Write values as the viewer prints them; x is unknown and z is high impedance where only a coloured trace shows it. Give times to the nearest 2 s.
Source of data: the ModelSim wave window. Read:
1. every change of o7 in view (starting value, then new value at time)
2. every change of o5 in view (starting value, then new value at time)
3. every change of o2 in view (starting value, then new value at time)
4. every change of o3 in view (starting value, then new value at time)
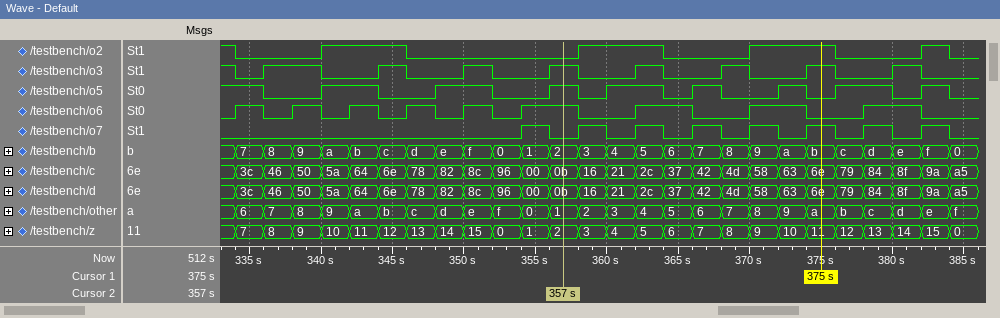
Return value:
0, 1 at 354 s, 0 at 356 s, 1 at 358 s, 0 at 360 s, 1 at 362 s, 0 at 364 s, 1 at 366 s, 0 at 368 s, 1 at 370 s, 0 at 372 s, 1 at 374 s, 0 at 376 s, 1 at 378 s, 0 at 380 s, 1 at 382 s, 0 at 384 s
1, 0 at 336 s, 1 at 340 s, 0 at 344 s, 1 at 348 s, 0 at 352 s, 1 at 356 s, 0 at 358 s, 1 at 360 s, 0 at 364 s, 1 at 366 s, 0 at 368 s, 1 at 372 s, 0 at 374 s, 1 at 376 s, 0 at 380 s, 1 at 382 s, 0 at 384 s
1, 0 at 334 s, 1 at 340 s, 0 at 346 s, 1 at 358 s, 0 at 364 s, 1 at 370 s, 0 at 376 s, 1 at 382 s, 0 at 384 s
1, 0 at 334 s, 1 at 336 s, 0 at 340 s, 1 at 344 s, 0 at 346 s, 1 at 350 s, 0 at 352 s, 1 at 356 s, 0 at 358 s, 1 at 362 s, 0 at 364 s, 1 at 368 s, 0 at 370 s, 1 at 374 s, 0 at 376 s, 1 at 380 s, 0 at 382 s
